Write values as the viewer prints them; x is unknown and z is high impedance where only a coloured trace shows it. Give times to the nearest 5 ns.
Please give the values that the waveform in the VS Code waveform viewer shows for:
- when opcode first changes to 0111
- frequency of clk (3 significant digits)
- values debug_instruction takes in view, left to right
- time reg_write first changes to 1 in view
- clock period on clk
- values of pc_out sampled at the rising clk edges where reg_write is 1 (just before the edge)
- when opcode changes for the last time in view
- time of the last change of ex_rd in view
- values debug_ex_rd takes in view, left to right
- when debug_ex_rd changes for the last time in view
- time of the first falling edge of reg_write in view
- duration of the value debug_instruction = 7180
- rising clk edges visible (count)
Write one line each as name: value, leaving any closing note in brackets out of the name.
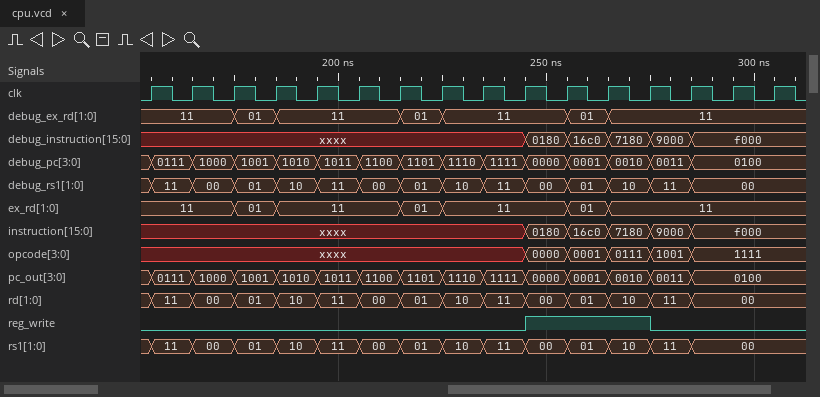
when opcode first changes to 0111: 265 ns
frequency of clk: 100 MHz
values debug_instruction takes in view, left to right: xxxx, 0180, 16c0, 7180, 9000, f000
time reg_write first changes to 1 in view: 245 ns
clock period on clk: 10 ns
values of pc_out sampled at the rising clk edges where reg_write is 1: 0000, 0001, 0010
when opcode changes for the last time in view: 285 ns
time of the last change of ex_rd in view: 265 ns
values debug_ex_rd takes in view, left to right: 11, 01, 11, 01, 11, 01, 11
when debug_ex_rd changes for the last time in view: 265 ns
time of the first falling edge of reg_write in view: 275 ns
duration of the value debug_instruction = 7180: 10 ns
rising clk edges visible: 16
